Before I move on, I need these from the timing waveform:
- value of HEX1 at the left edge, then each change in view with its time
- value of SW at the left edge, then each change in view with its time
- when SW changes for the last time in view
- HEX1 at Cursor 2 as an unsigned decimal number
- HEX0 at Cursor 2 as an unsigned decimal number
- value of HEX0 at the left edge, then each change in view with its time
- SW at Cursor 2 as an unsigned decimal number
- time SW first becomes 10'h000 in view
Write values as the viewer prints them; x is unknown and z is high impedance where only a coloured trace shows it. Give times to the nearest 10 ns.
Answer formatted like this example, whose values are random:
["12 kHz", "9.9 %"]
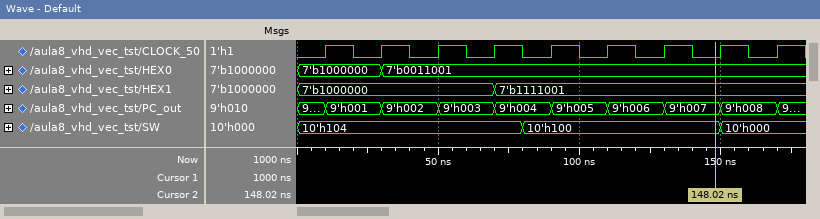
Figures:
["7'b1000000, 7'b1111001 at 70 ns", "10'h104, 10'h100 at 80 ns, 10'h000 at 150 ns", "150 ns", "121", "25", "7'b1000000, 7'b0011001 at 30 ns", "256", "150 ns"]
